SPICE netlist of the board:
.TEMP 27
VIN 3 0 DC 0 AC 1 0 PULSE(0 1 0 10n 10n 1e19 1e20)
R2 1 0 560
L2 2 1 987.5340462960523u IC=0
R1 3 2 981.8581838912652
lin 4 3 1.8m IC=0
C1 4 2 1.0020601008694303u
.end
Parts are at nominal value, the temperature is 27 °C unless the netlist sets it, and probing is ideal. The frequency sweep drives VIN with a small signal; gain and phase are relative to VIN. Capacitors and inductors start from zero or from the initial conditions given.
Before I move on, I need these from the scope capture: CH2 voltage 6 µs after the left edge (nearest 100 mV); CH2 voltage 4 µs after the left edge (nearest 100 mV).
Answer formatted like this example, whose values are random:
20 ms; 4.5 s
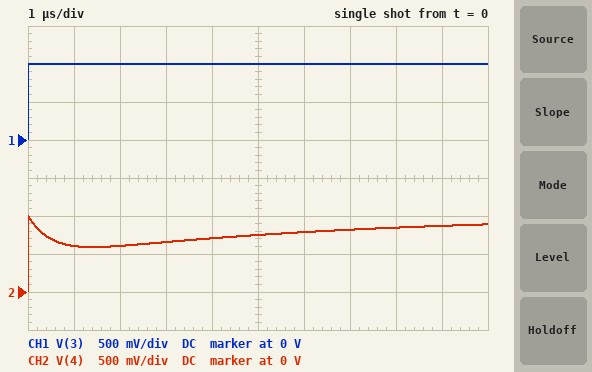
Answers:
800 mV; 700 mV
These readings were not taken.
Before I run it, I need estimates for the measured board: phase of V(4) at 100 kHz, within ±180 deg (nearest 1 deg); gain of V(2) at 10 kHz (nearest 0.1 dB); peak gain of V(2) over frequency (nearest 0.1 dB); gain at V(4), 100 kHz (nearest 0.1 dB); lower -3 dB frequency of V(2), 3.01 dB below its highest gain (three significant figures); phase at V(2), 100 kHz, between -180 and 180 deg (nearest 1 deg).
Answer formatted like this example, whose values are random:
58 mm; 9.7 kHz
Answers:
3 deg; -0.4 dB; 0 dB; -5.5 dB; 377 Hz; 3 deg
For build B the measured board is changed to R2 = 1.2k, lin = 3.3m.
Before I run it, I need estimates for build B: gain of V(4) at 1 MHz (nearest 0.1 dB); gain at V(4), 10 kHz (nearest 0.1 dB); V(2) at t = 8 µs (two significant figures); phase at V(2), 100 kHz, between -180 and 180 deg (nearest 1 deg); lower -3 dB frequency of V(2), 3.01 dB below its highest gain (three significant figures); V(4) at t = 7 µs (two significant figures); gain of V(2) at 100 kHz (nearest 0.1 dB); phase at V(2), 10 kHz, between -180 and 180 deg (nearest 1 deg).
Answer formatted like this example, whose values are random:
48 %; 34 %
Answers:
-0.4 dB; -0.4 dB; 870 mV; 1 deg; 184 Hz; 850 mV; -4.4 dB; -8 deg
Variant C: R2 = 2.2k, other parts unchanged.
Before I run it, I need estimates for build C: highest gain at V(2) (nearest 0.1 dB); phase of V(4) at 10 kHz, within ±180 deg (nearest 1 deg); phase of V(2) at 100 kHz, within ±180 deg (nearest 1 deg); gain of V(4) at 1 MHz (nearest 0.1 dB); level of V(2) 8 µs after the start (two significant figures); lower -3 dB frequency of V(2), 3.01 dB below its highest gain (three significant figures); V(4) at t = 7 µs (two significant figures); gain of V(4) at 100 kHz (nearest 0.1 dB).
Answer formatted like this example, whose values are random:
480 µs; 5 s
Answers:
0 dB; -3 deg; -6 deg; -0.6 dB; 980 mV; 49.0 Hz; 970 mV; -2.3 dB
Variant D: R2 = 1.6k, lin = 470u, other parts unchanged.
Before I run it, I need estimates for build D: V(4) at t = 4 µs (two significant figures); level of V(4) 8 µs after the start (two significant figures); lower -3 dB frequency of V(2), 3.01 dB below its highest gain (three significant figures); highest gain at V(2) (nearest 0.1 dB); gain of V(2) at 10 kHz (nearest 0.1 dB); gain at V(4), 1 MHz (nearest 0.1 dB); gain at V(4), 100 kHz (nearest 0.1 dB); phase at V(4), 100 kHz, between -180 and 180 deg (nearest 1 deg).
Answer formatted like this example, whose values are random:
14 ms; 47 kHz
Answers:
990 mV; 1.0 V; 126 Hz; 0 dB; 0 dB; -0.7 dB; -0.9 dB; -7 deg
